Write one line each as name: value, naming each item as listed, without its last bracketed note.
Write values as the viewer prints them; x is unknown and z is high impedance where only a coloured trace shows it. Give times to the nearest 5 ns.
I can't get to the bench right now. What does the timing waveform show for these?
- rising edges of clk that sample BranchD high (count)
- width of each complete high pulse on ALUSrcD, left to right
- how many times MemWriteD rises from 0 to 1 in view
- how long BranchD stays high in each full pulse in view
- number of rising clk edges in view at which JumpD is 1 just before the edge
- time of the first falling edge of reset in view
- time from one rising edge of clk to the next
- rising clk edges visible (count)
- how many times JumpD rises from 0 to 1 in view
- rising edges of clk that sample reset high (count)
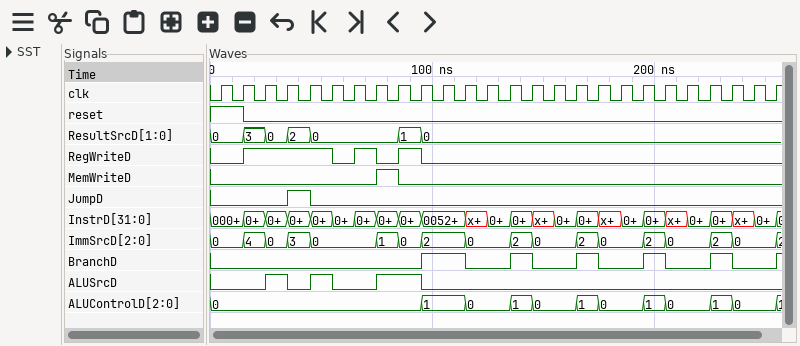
rising edges of clk that sample BranchD high: 6
width of each complete high pulse on ALUSrcD, left to right: 10 ns, 10 ns, 20 ns
how many times MemWriteD rises from 0 to 1 in view: 1
how long BranchD stays high in each full pulse in view: 20 ns, 10 ns, 10 ns, 10 ns, 10 ns
number of rising clk edges in view at which JumpD is 1 just before the edge: 1
time of the first falling edge of reset in view: 15 ns
time from one rising edge of clk to the next: 10 ns
rising clk edges visible: 26
how many times JumpD rises from 0 to 1 in view: 1
rising edges of clk that sample reset high: 2
